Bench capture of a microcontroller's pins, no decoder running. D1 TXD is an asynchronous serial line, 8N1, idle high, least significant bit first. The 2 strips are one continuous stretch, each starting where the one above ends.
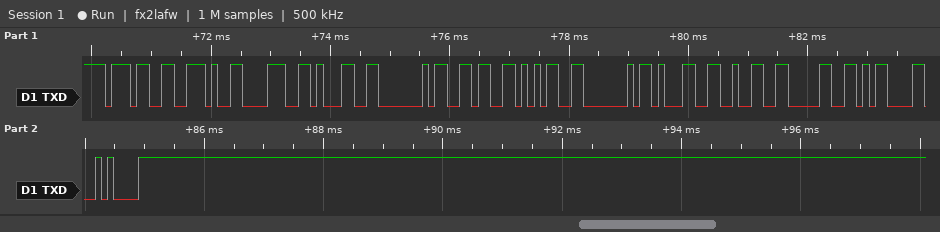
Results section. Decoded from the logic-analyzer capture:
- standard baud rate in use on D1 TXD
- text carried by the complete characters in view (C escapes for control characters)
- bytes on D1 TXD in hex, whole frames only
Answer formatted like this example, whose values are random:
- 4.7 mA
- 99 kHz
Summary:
- 9600 baud
- "7.81@65@120\r\n"
- 0x37 0x2E 0x38 0x31 0x40 0x36 0x35 0x40 0x31 0x32 0x30 0x0D 0x0A
